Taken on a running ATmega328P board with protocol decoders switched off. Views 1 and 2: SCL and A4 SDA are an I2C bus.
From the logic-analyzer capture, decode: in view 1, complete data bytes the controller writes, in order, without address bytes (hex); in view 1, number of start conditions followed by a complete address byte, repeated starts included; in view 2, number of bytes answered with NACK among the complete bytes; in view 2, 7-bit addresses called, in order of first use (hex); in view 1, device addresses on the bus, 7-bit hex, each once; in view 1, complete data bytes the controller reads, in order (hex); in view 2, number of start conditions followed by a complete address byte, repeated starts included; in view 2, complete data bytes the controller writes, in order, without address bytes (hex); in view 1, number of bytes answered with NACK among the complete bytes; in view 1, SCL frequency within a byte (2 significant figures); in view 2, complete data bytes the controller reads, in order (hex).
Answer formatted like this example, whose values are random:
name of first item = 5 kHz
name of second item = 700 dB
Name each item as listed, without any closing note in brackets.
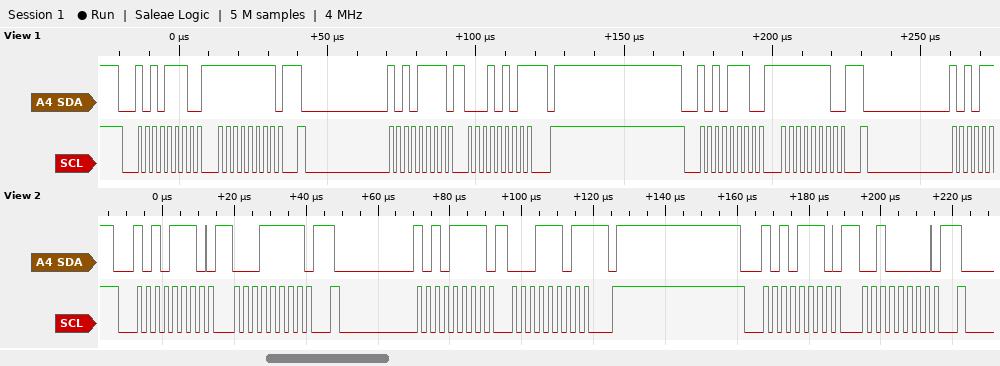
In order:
in view 1, complete data bytes the controller writes, in order, without address bytes = FF FE
in view 1, number of start conditions followed by a complete address byte, repeated starts included = 3
in view 2, number of bytes answered with NACK among the complete bytes = 1
in view 2, 7-bit addresses called, in order of first use = 0x57
in view 1, device addresses on the bus, 7-bit hex, each once = 0x57
in view 1, complete data bytes the controller reads, in order = 15
in view 2, number of start conditions followed by a complete address byte, repeated starts included = 3
in view 2, complete data bytes the controller writes, in order, without address bytes = 1F 20
in view 1, number of bytes answered with NACK among the complete bytes = 1
in view 1, SCL frequency within a byte = 400 kHz
in view 2, complete data bytes the controller reads, in order = 1D
